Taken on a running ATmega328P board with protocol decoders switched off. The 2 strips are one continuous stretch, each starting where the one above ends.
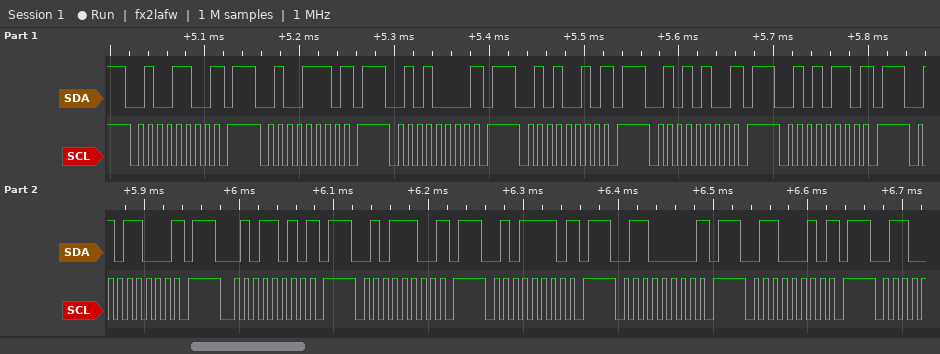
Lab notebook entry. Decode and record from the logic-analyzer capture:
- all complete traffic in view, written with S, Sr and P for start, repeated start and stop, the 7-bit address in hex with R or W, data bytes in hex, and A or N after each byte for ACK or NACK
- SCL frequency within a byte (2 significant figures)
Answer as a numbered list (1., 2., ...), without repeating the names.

1. S 26W N P S 27W N P S 28W N P S 29W N P S 2AW N P S 2BW N P S 2CW N P S 2DW N P S 2EW N P S 2FW N P S 30W N P S 31W N P
2. 100 kHz
